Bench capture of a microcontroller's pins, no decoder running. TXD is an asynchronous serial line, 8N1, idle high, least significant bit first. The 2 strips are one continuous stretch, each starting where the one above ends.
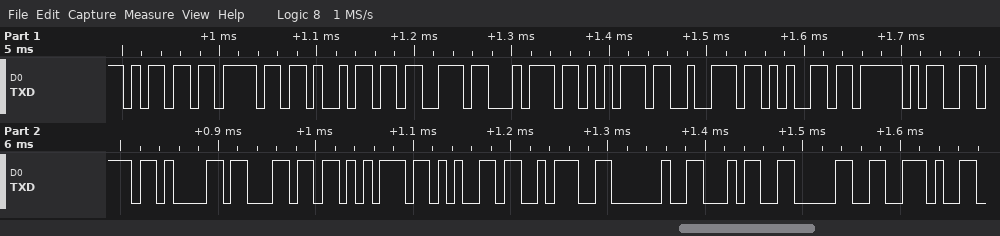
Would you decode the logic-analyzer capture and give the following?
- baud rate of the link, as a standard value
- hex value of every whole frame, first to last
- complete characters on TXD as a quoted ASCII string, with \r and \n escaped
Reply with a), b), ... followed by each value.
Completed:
a) 115200 baud
b) 6D 6F 69 73 74 75 72 65 5F 76 61 6C 75 65 3A 20 34 30 2E
c) "moisture_value: 40."
